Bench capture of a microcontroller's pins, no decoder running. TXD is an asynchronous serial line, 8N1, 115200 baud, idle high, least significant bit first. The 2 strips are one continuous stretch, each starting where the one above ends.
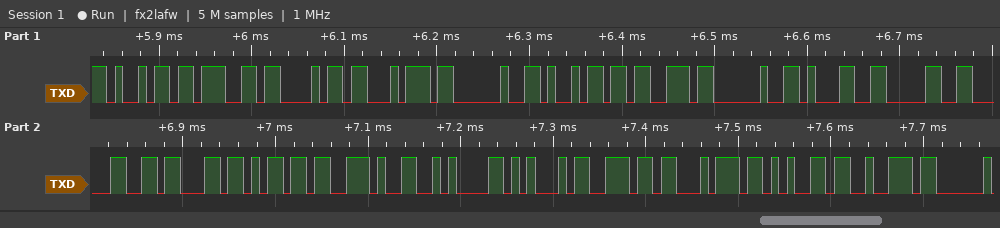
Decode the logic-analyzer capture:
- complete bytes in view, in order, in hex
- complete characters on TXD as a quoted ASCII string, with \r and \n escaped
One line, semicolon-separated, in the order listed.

0x69 0x67 0x68 0x74 0x20 0x69 0x73 0x20 0x31 0x30 0x30 0x63 0x6D 0x2E 0x0A 0x45 0x6E 0x74 0x65 0x72; "ight is 100cm.\nEnter"
